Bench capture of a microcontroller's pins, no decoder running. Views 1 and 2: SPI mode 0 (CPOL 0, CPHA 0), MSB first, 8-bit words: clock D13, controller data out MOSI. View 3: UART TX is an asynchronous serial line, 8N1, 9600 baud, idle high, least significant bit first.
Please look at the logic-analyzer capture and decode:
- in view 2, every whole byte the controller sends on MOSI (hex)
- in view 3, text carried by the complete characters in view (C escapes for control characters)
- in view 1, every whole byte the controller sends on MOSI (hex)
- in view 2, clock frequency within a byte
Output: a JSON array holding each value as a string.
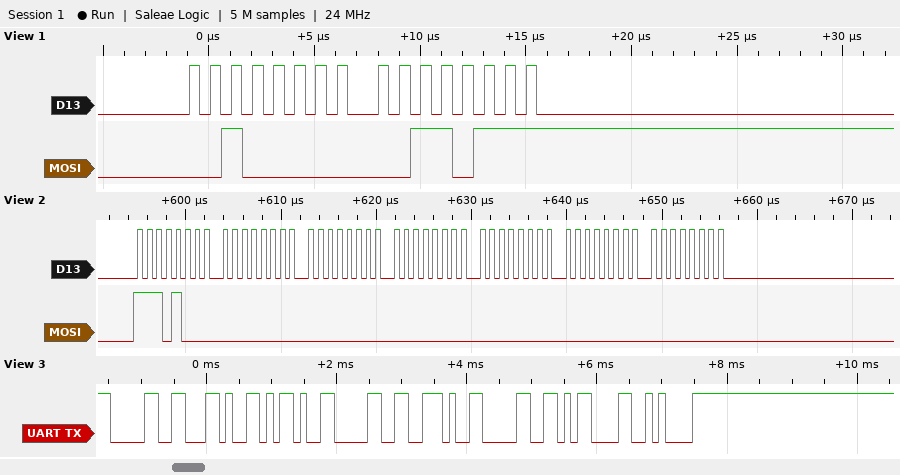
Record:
["E8 00 00 00 00 00 00", "\"0,-0.0\\r\\n\"", "0x20 0x37", "1 MHz"]
